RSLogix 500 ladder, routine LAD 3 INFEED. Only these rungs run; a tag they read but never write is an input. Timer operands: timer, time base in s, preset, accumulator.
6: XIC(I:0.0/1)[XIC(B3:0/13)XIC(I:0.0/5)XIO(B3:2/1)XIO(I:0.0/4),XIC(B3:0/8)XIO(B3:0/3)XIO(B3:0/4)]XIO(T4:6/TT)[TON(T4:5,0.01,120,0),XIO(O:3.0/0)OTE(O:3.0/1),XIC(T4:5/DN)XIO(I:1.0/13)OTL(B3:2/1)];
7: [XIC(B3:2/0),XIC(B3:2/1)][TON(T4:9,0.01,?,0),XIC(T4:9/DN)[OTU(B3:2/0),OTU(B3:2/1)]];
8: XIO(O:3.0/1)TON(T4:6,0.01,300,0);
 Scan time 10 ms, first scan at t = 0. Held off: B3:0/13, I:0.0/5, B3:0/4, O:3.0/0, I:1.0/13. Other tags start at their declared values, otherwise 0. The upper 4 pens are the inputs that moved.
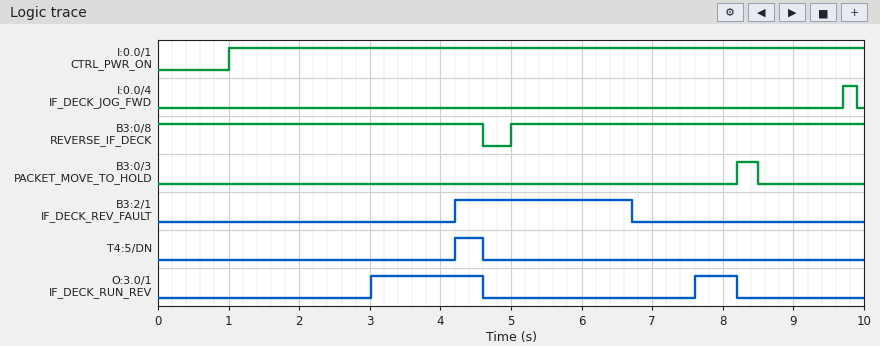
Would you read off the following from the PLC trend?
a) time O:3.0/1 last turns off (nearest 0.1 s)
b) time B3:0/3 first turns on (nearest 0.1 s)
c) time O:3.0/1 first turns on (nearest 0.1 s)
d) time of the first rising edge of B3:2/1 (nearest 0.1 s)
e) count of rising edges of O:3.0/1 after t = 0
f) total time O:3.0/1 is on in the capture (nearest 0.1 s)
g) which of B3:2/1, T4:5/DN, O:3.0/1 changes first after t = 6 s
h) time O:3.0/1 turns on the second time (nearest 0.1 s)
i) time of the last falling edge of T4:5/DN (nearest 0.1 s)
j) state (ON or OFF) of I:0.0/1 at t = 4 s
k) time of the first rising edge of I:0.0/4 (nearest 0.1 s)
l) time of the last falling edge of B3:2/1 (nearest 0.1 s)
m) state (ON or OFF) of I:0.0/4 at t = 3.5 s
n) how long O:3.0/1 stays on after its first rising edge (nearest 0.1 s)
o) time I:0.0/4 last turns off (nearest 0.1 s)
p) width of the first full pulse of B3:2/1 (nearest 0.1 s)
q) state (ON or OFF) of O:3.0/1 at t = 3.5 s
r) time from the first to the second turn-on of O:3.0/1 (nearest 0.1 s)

8.2 s
8.2 s
3.0 s
4.2 s
2
2.2 s
B3:2/1
7.6 s
4.6 s
ON
9.7 s
6.7 s
OFF
1.6 s
9.9 s
2.5 s
ON
4.6 s
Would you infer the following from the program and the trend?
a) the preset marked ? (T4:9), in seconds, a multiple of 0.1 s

2.5 s
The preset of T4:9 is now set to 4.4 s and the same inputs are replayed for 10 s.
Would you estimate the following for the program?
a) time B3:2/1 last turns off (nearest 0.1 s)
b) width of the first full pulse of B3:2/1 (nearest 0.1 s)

8.6 s
4.4 s
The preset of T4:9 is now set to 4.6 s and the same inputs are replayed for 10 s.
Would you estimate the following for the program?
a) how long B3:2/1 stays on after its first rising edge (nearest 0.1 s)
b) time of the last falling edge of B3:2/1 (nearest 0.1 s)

4.6 s
8.8 s
